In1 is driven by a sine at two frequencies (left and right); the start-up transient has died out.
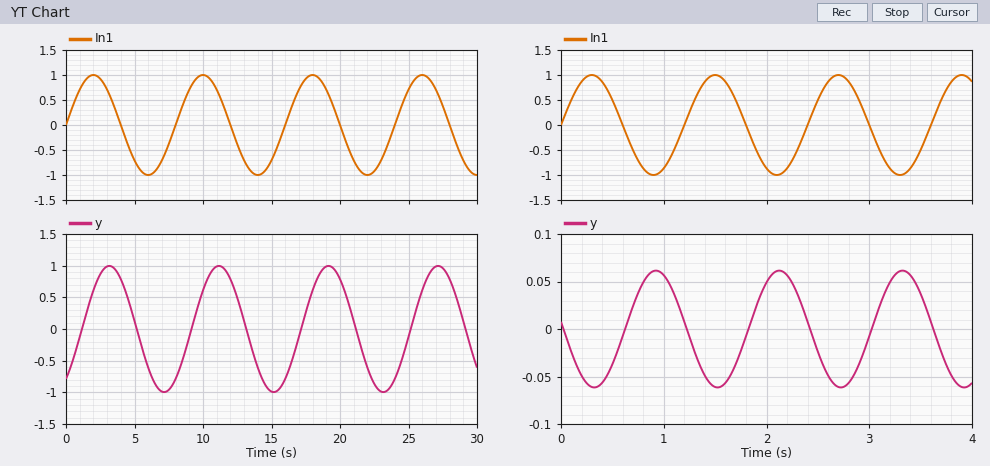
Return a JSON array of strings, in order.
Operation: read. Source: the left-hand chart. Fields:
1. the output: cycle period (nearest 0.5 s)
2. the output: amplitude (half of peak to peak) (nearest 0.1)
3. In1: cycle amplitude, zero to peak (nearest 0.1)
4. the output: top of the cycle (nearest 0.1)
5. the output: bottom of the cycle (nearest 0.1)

["8.0 s", "1.0", "1.0", "1.0", "-1.0"]
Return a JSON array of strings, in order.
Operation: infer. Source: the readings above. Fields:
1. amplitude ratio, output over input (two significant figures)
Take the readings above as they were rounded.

["1.0"]
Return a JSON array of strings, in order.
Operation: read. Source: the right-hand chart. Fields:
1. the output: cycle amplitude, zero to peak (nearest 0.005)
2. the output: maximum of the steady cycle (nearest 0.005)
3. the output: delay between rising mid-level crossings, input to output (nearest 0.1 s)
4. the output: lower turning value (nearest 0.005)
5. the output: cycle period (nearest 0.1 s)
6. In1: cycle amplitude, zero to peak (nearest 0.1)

["0.060", "0.060", "0.6 s", "-0.060", "1.2 s", "1.0"]
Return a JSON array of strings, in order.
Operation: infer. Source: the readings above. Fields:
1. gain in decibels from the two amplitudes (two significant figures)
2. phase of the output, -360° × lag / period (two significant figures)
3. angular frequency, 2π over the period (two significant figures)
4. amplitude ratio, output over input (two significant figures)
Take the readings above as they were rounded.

["-24 dB", "-180°", "5.2 rad/s", "0.060"]
